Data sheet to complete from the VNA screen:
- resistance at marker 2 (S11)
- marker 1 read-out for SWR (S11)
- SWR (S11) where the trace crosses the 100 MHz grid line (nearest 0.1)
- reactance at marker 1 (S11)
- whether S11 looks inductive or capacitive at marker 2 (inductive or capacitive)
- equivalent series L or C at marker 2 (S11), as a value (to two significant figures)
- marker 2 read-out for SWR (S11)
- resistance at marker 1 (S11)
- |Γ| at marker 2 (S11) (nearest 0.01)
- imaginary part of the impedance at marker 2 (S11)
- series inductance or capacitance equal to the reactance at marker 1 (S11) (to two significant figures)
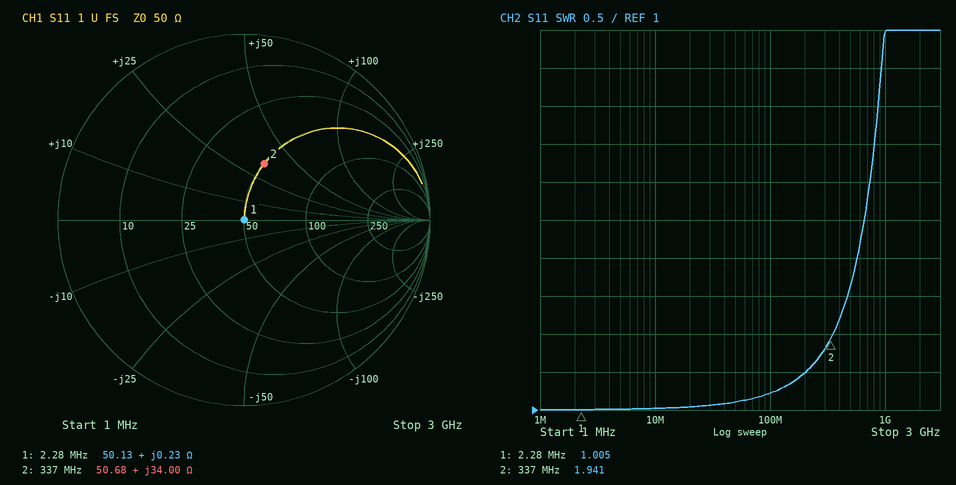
50.68 Ω
1.005
1.2
+0.23 Ω
inductive
16 nH
1.941
50.13 Ω
0.32
+34.00 Ω
16 nH
